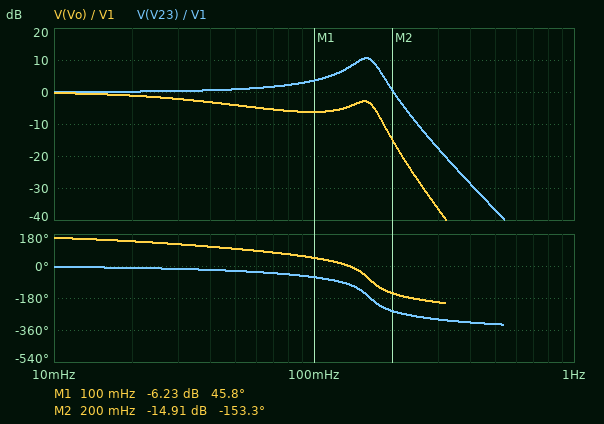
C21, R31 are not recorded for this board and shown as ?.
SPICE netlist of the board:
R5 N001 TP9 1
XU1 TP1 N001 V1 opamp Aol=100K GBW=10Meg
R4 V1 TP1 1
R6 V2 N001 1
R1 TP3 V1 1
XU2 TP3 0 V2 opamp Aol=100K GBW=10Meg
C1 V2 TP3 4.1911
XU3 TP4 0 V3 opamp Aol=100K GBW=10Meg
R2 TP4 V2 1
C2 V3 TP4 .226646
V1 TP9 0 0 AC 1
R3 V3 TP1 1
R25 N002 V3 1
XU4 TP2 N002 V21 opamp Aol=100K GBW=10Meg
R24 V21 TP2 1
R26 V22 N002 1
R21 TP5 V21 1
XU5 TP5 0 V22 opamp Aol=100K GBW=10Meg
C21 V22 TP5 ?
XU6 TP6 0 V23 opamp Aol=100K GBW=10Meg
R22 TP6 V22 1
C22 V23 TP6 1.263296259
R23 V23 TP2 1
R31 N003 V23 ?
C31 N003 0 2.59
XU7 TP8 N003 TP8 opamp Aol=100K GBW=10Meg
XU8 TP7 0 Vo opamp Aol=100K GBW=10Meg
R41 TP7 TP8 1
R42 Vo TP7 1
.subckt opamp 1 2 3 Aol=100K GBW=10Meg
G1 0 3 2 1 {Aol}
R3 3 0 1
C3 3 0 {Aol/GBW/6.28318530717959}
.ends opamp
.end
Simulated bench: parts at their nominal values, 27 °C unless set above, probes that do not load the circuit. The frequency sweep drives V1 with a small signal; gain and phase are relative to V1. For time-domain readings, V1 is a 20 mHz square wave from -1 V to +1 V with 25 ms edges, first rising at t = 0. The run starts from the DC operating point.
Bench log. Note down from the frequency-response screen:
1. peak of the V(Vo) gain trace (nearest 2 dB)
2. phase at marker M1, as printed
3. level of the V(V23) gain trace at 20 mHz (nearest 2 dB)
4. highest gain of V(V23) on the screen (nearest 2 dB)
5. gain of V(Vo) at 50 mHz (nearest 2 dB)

0 dB
45.8 deg
0 dB
10 dB
-4 dB
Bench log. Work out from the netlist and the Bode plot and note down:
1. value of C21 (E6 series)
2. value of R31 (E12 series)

680 mF
1.8 Ω
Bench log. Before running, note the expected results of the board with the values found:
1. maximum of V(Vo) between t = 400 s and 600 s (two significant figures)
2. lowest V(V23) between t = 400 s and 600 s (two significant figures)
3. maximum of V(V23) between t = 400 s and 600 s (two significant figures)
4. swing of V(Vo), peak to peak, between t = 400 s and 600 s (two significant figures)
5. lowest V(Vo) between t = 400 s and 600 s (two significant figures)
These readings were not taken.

1.0 V
-2.1 V
2.1 V
2.0 V
-1.0 V
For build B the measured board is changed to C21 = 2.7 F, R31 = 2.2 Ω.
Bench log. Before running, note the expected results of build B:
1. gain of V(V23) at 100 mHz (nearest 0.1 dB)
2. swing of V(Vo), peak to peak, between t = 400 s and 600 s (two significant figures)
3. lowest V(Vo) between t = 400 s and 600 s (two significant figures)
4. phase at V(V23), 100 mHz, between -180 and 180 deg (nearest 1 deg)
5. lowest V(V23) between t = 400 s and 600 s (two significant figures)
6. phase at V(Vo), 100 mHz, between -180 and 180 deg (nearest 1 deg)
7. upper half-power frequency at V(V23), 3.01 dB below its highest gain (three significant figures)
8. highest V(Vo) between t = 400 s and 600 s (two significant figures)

5.1 dB
2.0 V
-980 mV
-126 deg
-2.2 V
-21 deg
165 mHz
980 mV
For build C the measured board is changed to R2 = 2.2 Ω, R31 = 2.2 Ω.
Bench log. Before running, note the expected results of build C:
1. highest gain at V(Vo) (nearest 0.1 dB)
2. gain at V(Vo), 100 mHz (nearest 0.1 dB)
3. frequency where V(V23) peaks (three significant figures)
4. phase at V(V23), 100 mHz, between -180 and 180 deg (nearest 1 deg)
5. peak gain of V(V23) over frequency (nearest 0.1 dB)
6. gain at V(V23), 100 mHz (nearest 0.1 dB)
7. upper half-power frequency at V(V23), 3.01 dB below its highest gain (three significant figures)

0 dB
-2.8 dB
106 mHz
-111 deg
9.0 dB
8.6 dB
123 mHz
